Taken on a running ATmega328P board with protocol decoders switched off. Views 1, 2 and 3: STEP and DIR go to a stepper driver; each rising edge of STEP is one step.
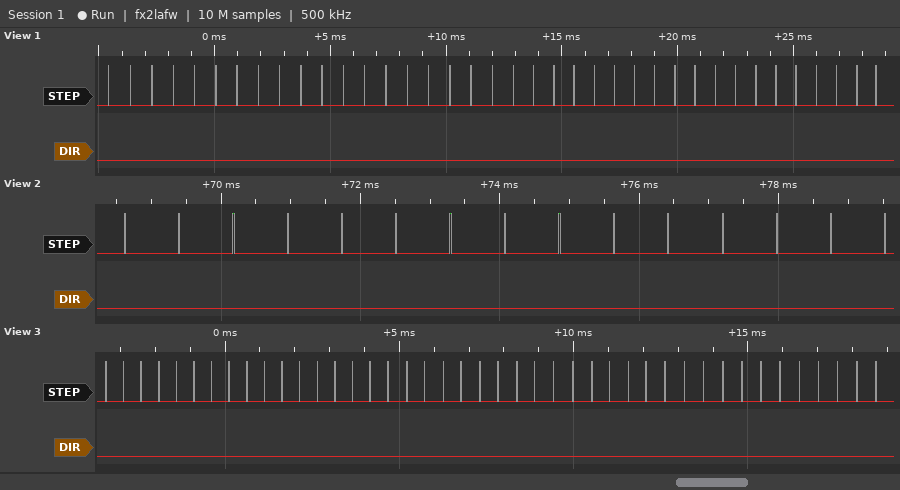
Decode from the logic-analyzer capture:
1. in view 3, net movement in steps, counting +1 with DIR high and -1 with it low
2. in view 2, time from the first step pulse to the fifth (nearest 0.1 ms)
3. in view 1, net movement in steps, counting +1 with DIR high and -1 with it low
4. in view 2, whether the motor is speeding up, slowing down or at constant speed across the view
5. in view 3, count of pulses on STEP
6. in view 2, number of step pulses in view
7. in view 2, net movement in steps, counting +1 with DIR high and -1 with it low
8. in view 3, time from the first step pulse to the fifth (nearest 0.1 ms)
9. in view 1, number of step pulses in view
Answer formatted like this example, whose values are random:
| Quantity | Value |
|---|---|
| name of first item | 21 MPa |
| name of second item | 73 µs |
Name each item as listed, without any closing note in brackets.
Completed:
| Quantity | Value |
|---|---|
| in view 3, net movement in steps, counting +1 with DIR high and -1 with it low | -43 |
| in view 2, time from the first step pulse to the fifth | 3.1 ms |
| in view 1, net movement in steps, counting +1 with DIR high and -1 with it low | -38 |
| in view 2, whether the motor is speeding up, slowing down or at constant speed across the view | constant speed |
| in view 3, count of pulses on STEP | 43 |
| in view 2, number of step pulses in view | 15 |
| in view 2, net movement in steps, counting +1 with DIR high and -1 with it low | -15 |
| in view 3, time from the first step pulse to the fifth | 2.0 ms |
| in view 1, number of step pulses in view | 38 |
